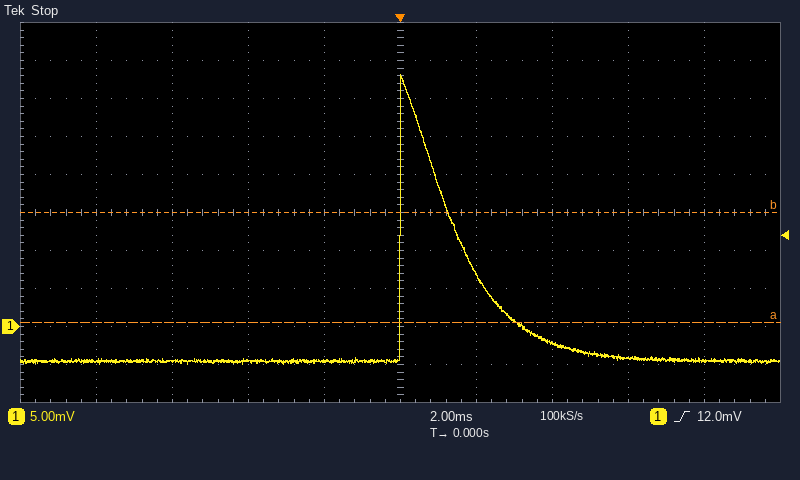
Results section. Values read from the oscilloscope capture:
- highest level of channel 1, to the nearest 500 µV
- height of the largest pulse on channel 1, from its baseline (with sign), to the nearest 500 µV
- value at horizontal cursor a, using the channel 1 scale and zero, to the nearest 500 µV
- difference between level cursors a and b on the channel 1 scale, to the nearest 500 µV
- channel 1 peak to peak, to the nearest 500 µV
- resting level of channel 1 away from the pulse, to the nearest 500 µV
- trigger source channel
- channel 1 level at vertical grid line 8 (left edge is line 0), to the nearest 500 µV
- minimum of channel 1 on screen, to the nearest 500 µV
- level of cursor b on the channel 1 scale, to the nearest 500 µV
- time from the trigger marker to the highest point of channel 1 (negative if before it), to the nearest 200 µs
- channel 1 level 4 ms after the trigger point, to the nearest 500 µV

33.0 mV
+37.5 mV
500 µV
14.5 mV
38.0 mV
-4.5 mV
channel 1
-4.0 mV
-5.0 mV
15.0 mV
0.0 ms
-2.0 mV
